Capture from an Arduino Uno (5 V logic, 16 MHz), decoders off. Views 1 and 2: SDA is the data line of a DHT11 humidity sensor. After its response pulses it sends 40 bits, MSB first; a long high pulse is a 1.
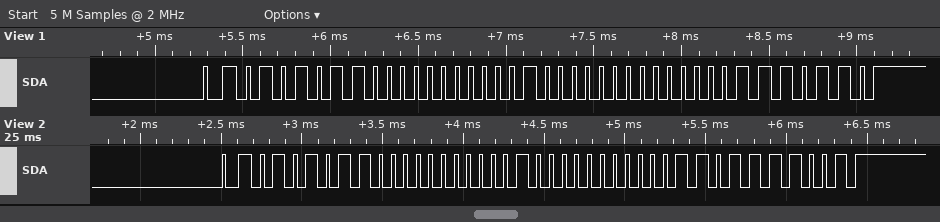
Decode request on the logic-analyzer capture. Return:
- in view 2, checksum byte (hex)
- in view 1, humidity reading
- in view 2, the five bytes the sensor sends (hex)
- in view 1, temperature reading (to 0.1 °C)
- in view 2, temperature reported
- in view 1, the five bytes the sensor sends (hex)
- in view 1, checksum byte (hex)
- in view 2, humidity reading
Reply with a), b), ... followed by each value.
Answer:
a) 0x79
b) 86 %
c) 56 00 20 03 79
d) 32.0 °C
e) 32.3 °C
f) 56 00 20 00 76
g) 0x76
h) 86 %
